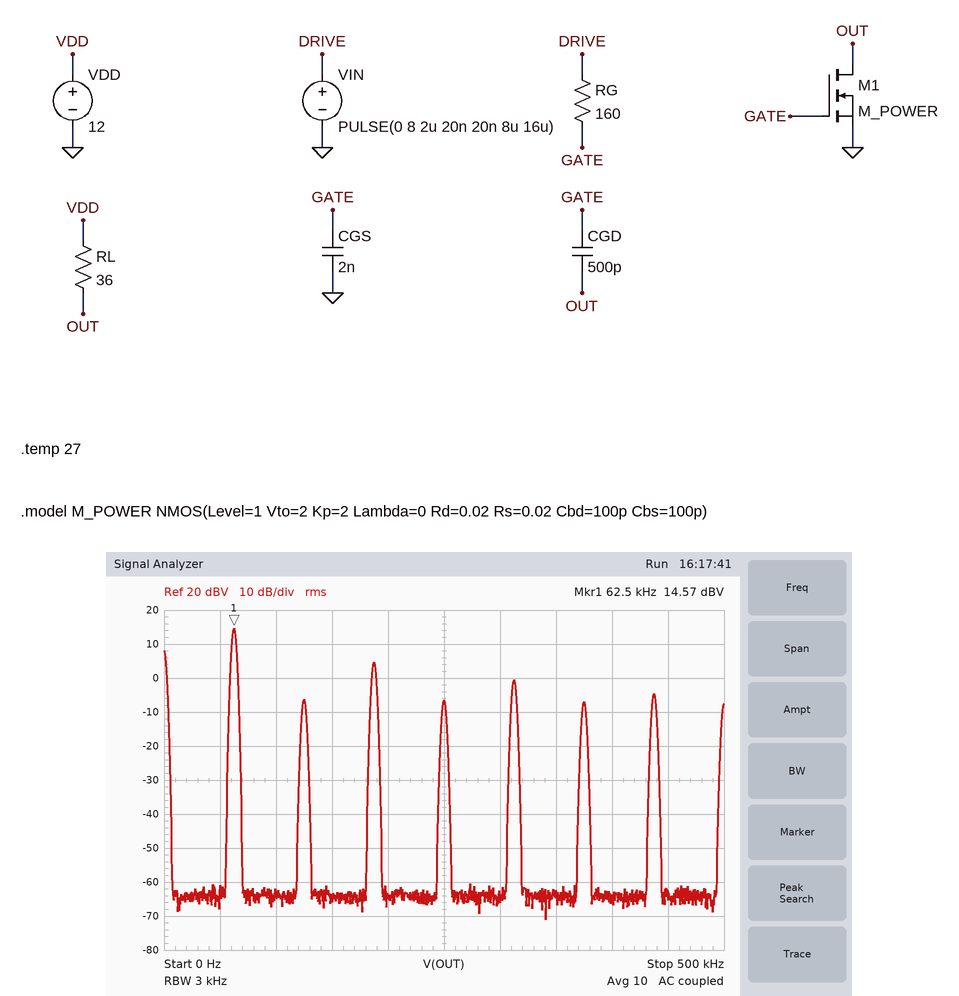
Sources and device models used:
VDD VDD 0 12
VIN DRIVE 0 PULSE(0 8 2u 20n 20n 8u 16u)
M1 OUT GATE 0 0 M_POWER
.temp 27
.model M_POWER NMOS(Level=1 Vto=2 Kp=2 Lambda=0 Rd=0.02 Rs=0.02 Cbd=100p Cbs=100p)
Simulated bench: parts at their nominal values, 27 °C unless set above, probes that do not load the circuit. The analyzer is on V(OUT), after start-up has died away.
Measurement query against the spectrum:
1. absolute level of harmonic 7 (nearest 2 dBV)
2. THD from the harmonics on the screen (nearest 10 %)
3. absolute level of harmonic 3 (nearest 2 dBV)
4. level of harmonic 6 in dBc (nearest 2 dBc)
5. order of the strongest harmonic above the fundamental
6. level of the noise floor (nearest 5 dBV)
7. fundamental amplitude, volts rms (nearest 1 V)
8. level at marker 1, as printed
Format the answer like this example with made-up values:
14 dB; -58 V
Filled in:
-4 dBV; 40 %; 4 dBV; -22 dBc; 3; -65 dBV; 5 V; 14.57 dBV
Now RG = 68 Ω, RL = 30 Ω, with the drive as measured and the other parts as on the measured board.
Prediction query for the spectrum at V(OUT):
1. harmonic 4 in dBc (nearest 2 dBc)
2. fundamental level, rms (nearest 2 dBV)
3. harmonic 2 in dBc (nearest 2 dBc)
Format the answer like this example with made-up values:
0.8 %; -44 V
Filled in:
-28 dBc; 14 dBV; -28 dBc
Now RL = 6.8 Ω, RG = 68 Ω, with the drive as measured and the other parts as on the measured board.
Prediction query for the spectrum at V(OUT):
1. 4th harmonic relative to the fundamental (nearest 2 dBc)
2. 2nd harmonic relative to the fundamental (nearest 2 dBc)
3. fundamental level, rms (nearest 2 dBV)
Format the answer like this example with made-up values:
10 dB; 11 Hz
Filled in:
-32 dBc; -32 dBc; 14 dBV
